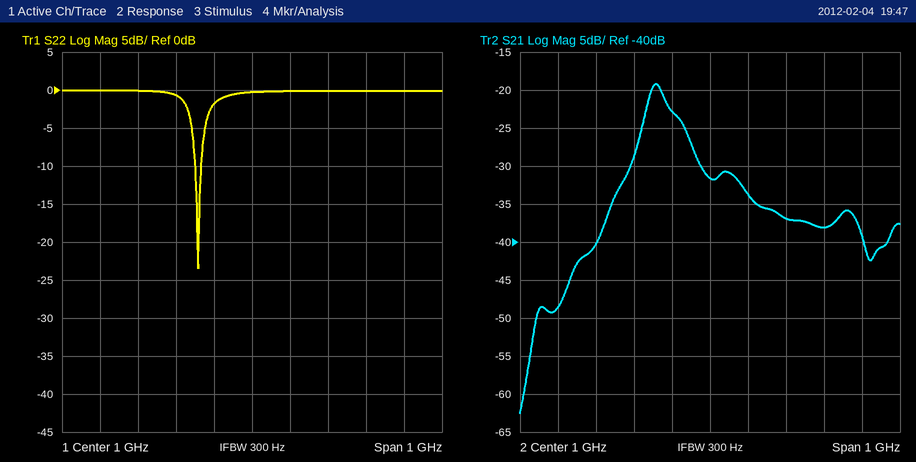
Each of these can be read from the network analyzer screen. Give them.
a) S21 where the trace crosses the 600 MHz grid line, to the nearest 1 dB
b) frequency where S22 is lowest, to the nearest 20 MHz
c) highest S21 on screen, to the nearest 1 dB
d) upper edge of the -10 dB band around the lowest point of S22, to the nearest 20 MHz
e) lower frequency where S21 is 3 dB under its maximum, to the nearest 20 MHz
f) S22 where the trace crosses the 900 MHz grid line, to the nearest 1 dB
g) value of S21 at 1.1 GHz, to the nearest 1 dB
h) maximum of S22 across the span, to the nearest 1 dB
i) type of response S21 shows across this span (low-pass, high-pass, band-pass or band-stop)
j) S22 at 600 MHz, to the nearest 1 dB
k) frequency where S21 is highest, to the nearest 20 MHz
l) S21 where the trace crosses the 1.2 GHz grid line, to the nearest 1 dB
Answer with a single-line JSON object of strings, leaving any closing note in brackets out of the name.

{"S21 where the trace crosses the 600 MHz grid line, to the nearest 1 dB": "-49 dB", "frequency where S22 is lowest, to the nearest 20 MHz": "860 MHz", "highest S21 on screen, to the nearest 1 dB": "-19 dB", "upper edge of the -10 dB band around the lowest point of S22, to the nearest 20 MHz": "860 MHz", "lower frequency where S21 is 3 dB under its maximum, to the nearest 20 MHz": "840 MHz", "S22 where the trace crosses the 900 MHz grid line, to the nearest 1 dB": "-2 dB", "value of S21 at 1.1 GHz, to the nearest 1 dB": "-34 dB", "maximum of S22 across the span, to the nearest 1 dB": "0 dB", "type of response S21 shows across this span": "band-pass", "S22 at 600 MHz, to the nearest 1 dB": "0 dB", "frequency where S21 is highest, to the nearest 20 MHz": "860 MHz", "S21 where the trace crosses the 1.2 GHz grid line, to the nearest 1 dB": "-37 dB"}
